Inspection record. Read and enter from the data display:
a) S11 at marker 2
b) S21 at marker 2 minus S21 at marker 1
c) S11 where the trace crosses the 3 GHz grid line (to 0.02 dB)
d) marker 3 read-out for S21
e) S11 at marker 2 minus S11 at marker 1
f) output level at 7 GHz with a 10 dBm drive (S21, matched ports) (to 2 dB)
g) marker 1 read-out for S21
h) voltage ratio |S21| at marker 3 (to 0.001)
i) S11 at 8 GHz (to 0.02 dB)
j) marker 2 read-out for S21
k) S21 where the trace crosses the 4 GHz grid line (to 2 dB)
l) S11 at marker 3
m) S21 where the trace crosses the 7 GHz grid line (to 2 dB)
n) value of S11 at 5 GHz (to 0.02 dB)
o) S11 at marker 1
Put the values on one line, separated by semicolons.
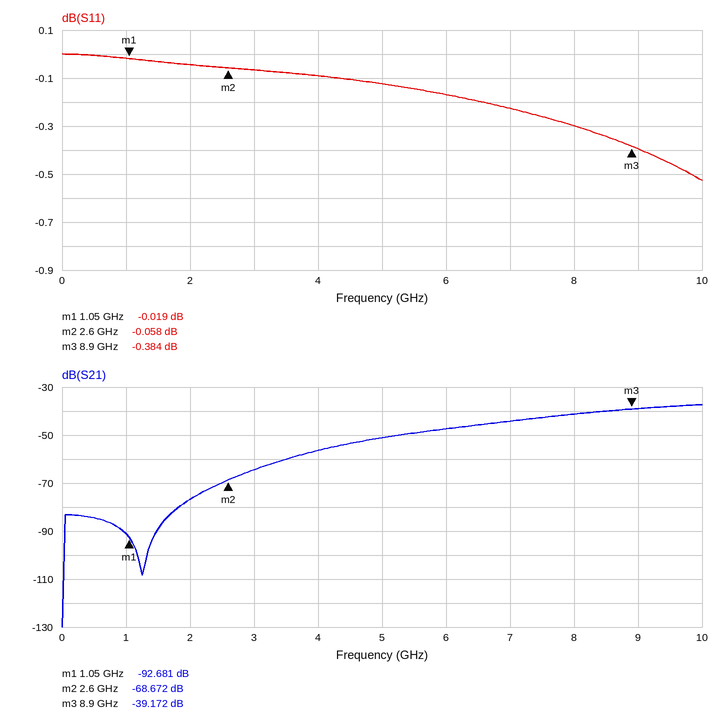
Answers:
-0.058 dB; 24.009 dB; -0.06 dB; -39.172 dB; -0.039 dB; -34 dBm; -92.681 dB; 0.011; -0.30 dB; -68.672 dB; -56 dB; -0.384 dB; -44 dB; -0.12 dB; -0.019 dB
